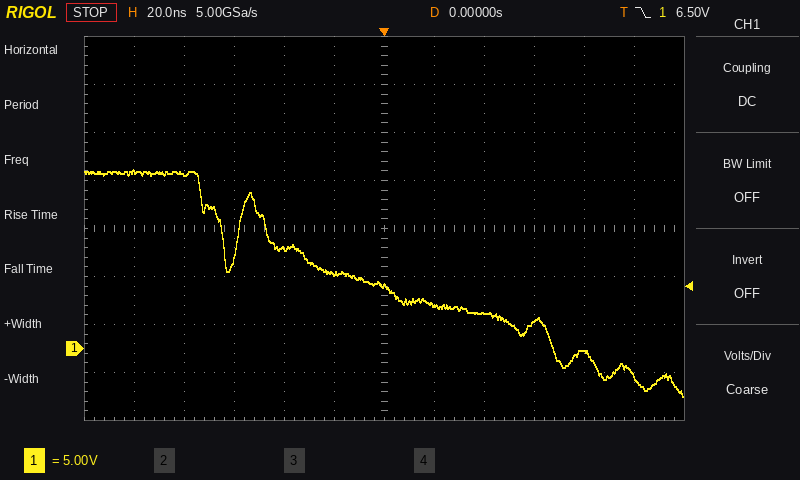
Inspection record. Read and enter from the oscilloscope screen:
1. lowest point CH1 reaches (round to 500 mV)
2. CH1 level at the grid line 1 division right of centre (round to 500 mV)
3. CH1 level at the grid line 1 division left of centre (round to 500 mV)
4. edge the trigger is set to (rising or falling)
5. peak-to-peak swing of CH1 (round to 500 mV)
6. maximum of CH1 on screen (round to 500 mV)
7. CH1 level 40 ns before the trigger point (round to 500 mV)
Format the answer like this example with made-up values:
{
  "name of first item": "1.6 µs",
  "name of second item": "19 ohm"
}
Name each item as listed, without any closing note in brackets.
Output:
{
  "lowest point CH1 reaches": "-5.0 V",
  "CH1 level at the grid line 1 division right of centre": "4.5 V",
  "CH1 level at the grid line 1 division left of centre": "8.0 V",
  "edge the trigger is set to": "falling",
  "peak-to-peak swing of CH1": "23.5 V",
  "maximum of CH1 on screen": "18.5 V",
  "CH1 level 40 ns before the trigger point": "10.5 V"
}
